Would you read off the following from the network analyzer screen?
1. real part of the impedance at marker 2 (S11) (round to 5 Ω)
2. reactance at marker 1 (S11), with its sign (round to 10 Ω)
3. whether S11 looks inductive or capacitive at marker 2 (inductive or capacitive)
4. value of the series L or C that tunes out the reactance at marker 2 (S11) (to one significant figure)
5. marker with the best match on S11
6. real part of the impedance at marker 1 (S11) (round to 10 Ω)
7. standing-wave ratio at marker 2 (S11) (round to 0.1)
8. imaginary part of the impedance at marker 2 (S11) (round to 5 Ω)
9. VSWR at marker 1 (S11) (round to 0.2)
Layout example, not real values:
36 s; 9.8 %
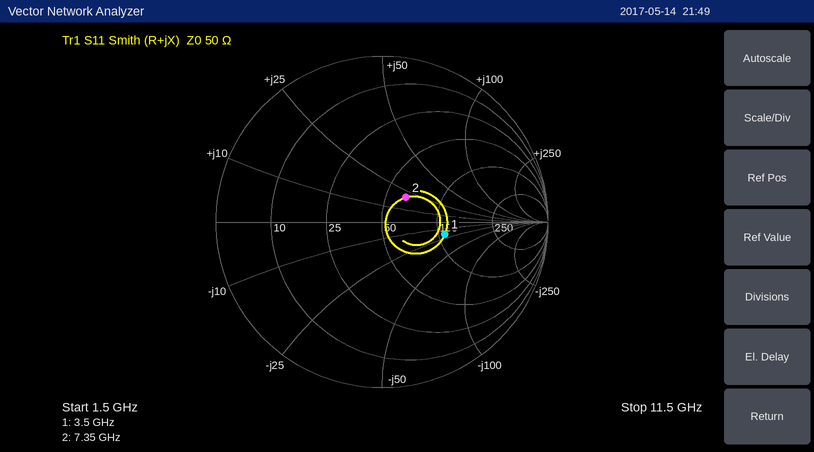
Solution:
65 Ω; -20 Ω; inductive; 1 pF; marker 2; 110 Ω; 1.5; +20 Ω; 2.2
